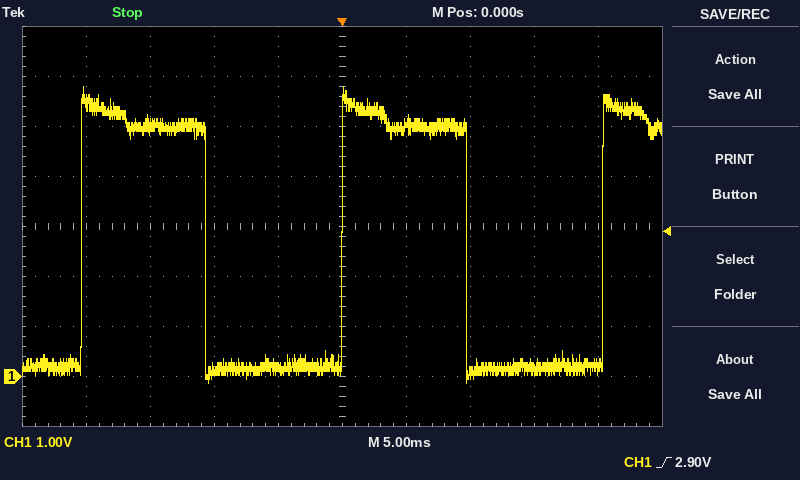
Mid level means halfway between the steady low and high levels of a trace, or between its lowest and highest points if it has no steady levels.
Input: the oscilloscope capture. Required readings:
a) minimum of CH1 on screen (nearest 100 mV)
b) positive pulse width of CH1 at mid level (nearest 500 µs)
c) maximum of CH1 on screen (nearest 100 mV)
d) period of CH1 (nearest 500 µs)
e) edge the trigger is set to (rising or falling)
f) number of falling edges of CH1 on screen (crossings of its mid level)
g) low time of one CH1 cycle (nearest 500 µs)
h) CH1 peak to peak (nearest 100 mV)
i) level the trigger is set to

-100 mV
9.5 ms
5.8 V
20.5 ms
rising
2
10.5 ms
5.9 V
2.90 V
